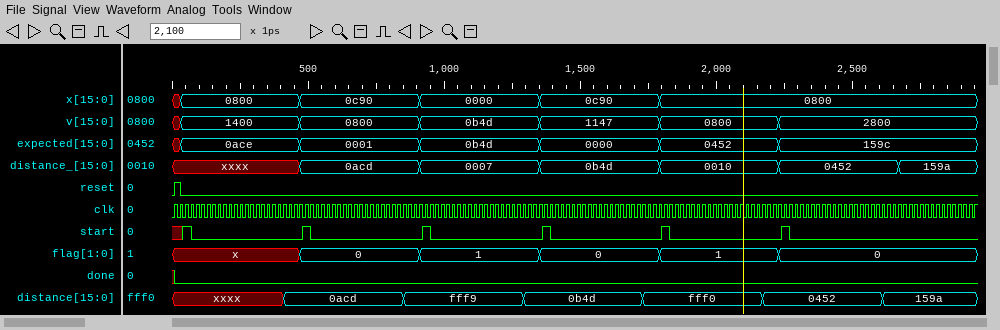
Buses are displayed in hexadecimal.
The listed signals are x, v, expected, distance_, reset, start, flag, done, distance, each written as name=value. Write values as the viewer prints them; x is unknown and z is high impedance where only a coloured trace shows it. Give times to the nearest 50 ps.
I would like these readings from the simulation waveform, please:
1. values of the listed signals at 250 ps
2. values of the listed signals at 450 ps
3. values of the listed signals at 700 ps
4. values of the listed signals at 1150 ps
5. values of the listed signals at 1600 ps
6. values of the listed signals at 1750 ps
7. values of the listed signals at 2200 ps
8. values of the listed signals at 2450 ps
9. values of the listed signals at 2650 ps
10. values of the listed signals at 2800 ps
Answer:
x=0800, v=1400, expected=0ace, distance_=xxxx, reset=0, start=0, flag=x, done=0, distance=xxxx
x=0800, v=1400, expected=0ace, distance_=xxxx, reset=0, start=0, flag=x, done=0, distance=0acd
x=0c90, v=0800, expected=0001, distance_=0acd, reset=0, start=0, flag=0, done=0, distance=0acd
x=0000, v=0b4d, expected=0b4d, distance_=0007, reset=0, start=0, flag=1, done=0, distance=fff9
x=0c90, v=1147, expected=0000, distance_=0b4d, reset=0, start=0, flag=0, done=0, distance=0b4d
x=0c90, v=1147, expected=0000, distance_=0b4d, reset=0, start=0, flag=0, done=0, distance=fff0
x=0800, v=0800, expected=0452, distance_=0010, reset=0, start=0, flag=1, done=0, distance=0452
x=0800, v=2800, expected=159c, distance_=0452, reset=0, start=0, flag=0, done=0, distance=0452
x=0800, v=2800, expected=159c, distance_=0452, reset=0, start=0, flag=0, done=0, distance=159a
x=0800, v=2800, expected=159c, distance_=159a, reset=0, start=0, flag=0, done=0, distance=159a
